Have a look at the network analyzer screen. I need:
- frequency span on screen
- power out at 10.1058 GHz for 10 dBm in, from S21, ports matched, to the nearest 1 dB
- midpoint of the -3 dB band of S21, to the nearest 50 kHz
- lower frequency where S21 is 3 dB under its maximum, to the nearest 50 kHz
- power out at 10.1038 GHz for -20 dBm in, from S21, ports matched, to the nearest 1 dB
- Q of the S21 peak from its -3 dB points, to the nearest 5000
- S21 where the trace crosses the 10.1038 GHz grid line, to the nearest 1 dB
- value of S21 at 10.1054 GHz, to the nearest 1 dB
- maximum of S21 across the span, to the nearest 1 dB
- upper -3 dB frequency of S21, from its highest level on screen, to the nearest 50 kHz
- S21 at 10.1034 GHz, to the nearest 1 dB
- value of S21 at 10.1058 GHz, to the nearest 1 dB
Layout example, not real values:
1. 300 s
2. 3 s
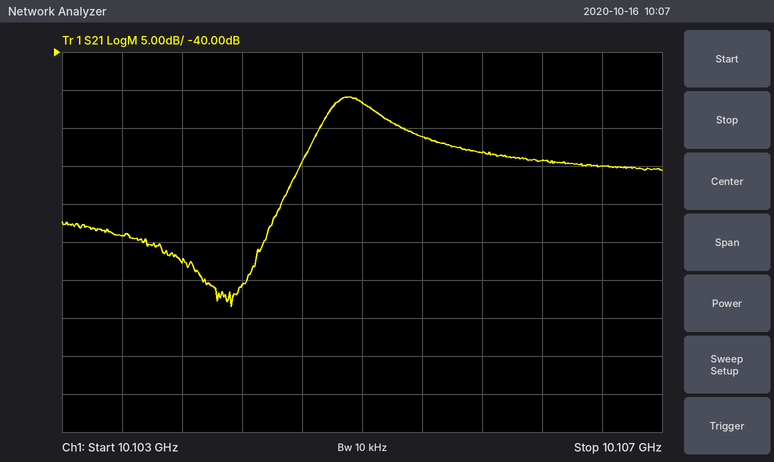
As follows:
1. 4 MHz
2. -43 dBm
3. 10.10495 GHz
4. 10.10475 GHz
5. -88 dBm
6. 25000
7. -68 dB
8. -51 dB
9. -46 dB
10. 10.10515 GHz
11. -64 dB
12. -53 dB
